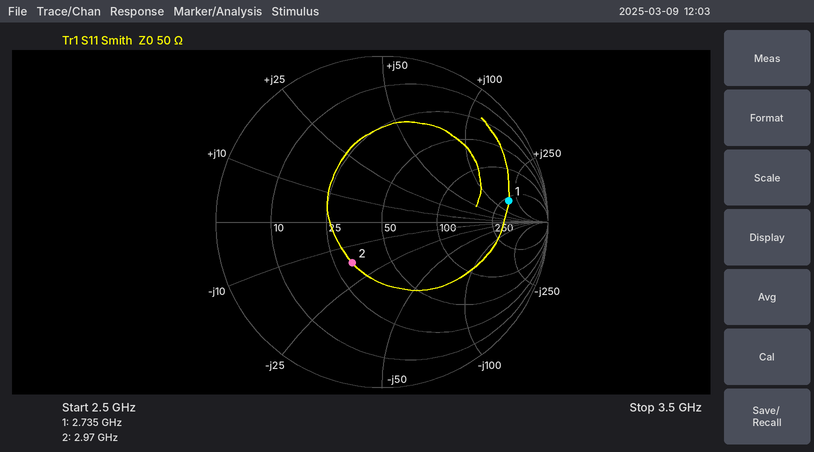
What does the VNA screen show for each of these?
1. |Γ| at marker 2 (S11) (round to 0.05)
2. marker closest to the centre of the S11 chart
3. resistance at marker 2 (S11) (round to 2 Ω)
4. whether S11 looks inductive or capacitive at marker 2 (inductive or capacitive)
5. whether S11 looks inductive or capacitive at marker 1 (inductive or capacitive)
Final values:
0.30
marker 2
32 Ω
capacitive
inductive
